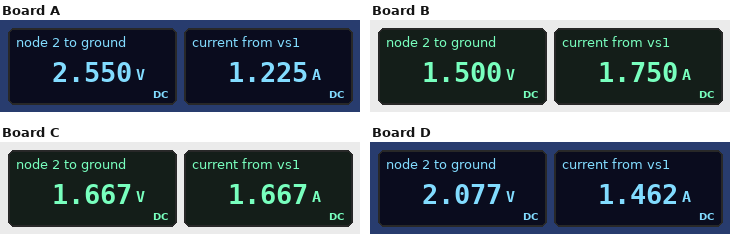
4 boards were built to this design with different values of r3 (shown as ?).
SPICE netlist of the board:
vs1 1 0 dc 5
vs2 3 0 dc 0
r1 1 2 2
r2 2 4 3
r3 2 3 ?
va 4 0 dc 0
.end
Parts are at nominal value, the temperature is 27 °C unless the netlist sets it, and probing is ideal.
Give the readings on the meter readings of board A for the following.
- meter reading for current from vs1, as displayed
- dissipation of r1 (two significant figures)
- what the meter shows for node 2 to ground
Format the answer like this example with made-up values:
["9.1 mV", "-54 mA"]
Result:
["1.225 A", "3.0 W", "2.550 V"]
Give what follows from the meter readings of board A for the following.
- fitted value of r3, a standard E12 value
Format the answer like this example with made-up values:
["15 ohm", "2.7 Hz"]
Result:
["6.8 Ω"]
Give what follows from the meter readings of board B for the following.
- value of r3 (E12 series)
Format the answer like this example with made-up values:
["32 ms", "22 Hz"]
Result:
["1.2 Ω"]
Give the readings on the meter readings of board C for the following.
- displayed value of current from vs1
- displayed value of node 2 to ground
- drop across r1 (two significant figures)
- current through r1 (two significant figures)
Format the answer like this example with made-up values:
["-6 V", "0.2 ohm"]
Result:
["1.667 A", "1.667 V", "3.3 V", "1.7 A"]
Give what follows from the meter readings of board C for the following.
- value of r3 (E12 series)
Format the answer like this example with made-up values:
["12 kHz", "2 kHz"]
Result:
["1.5 Ω"]
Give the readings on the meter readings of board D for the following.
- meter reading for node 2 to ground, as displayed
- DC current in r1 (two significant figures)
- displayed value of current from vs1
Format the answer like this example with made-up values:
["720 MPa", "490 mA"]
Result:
["2.077 V", "1.5 A", "1.462 A"]
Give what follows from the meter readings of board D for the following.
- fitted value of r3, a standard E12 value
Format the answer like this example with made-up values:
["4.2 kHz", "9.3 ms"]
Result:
["2.7 Ω"]
